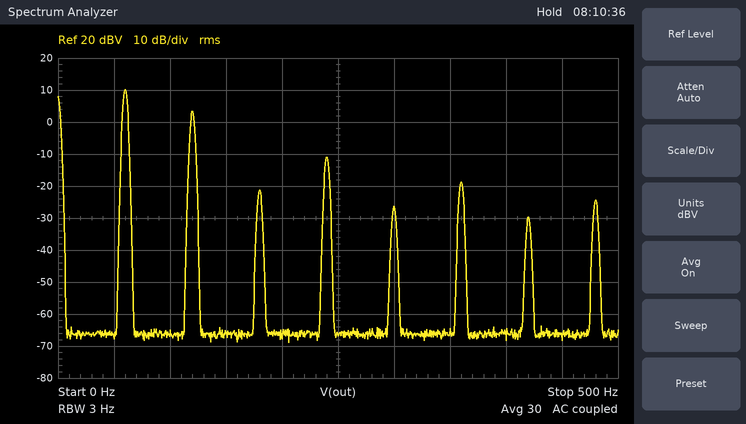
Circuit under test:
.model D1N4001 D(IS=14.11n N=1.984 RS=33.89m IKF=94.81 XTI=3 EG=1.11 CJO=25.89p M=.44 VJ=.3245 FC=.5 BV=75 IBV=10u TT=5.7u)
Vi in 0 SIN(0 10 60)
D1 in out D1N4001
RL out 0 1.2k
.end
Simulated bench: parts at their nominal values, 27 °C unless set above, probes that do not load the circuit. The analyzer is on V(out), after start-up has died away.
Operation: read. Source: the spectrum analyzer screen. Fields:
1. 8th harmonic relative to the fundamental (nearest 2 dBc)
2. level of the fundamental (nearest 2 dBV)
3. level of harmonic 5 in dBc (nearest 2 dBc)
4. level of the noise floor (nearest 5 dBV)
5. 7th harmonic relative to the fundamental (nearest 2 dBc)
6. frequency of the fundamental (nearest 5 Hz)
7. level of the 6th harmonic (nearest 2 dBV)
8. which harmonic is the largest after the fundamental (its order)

-34 dBc
10 dBV
-36 dBc
-65 dBV
-40 dBc
60 Hz
-18 dBV
2
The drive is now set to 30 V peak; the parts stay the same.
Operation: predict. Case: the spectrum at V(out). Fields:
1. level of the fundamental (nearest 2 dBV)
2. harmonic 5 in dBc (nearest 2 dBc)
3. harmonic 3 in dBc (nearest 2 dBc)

20 dBV
-46 dBc
-40 dBc
